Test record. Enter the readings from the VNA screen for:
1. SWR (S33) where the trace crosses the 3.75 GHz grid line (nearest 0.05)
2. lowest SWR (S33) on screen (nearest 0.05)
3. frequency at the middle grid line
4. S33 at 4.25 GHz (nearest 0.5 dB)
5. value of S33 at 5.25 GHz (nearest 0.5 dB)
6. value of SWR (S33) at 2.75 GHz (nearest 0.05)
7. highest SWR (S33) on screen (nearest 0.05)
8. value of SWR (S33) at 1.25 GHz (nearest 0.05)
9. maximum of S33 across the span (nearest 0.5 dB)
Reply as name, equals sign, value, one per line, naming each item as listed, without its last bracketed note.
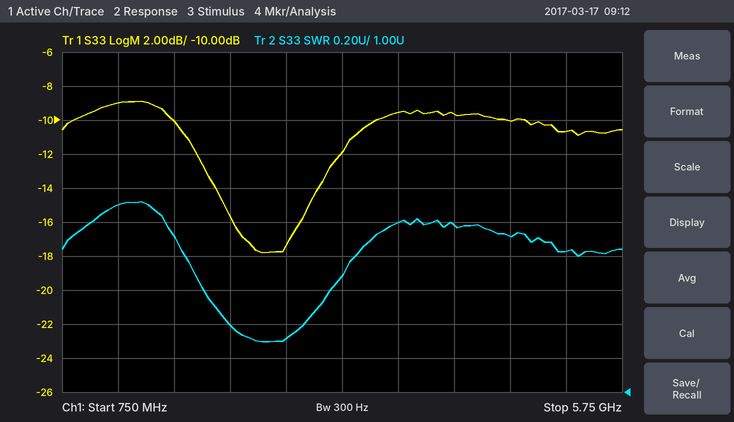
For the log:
SWR (S33) where the trace crosses the 3.75 GHz grid line = 2.00
lowest SWR (S33) on screen = 1.30
frequency at the middle grid line = 3.25 GHz
S33 at 4.25 GHz = -9.5 dB
value of S33 at 5.25 GHz = -10.5 dB
value of SWR (S33) at 2.75 GHz = 1.30
highest SWR (S33) on screen = 2.10
value of SWR (S33) at 1.25 GHz = 2.10
maximum of S33 across the span = -9.0 dB
